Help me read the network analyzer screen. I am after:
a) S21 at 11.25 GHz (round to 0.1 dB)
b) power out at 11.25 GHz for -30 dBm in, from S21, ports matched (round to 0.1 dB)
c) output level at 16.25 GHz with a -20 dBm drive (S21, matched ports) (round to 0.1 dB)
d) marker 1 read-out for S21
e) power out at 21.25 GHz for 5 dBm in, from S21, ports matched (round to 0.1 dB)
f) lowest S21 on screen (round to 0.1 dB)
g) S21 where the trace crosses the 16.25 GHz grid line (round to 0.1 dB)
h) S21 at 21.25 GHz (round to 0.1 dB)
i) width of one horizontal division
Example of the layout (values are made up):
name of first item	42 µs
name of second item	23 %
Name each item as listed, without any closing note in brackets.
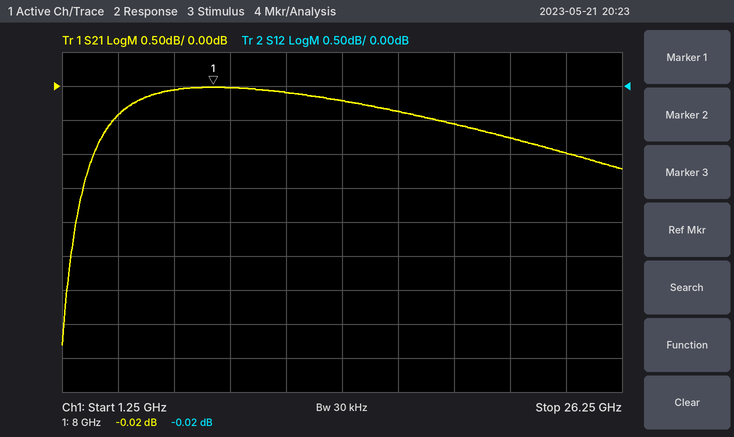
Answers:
S21 at 11.25 GHz	-0.1 dB
power out at 11.25 GHz for -30 dBm in, from S21, ports matched	-30.1 dBm
output level at 16.25 GHz with a -20 dBm drive (S21, matched ports)	-20.4 dBm
marker 1 read-out for S21	-0.02 dB
power out at 21.25 GHz for 5 dBm in, from S21, ports matched	4.2 dBm
lowest S21 on screen	-3.8 dB
S21 where the trace crosses the 16.25 GHz grid line	-0.4 dB
S21 at 21.25 GHz	-0.8 dB
width of one horizontal division	2.5 GHz
